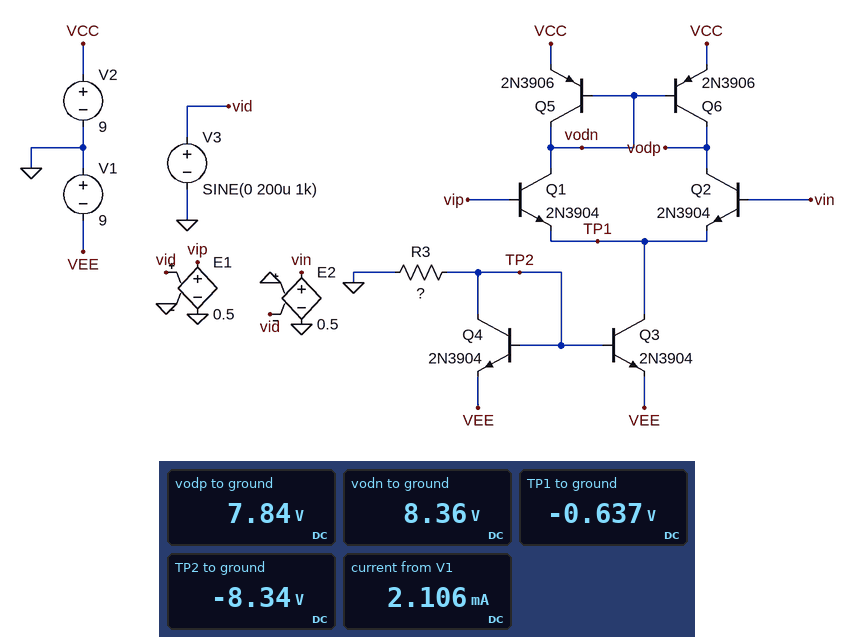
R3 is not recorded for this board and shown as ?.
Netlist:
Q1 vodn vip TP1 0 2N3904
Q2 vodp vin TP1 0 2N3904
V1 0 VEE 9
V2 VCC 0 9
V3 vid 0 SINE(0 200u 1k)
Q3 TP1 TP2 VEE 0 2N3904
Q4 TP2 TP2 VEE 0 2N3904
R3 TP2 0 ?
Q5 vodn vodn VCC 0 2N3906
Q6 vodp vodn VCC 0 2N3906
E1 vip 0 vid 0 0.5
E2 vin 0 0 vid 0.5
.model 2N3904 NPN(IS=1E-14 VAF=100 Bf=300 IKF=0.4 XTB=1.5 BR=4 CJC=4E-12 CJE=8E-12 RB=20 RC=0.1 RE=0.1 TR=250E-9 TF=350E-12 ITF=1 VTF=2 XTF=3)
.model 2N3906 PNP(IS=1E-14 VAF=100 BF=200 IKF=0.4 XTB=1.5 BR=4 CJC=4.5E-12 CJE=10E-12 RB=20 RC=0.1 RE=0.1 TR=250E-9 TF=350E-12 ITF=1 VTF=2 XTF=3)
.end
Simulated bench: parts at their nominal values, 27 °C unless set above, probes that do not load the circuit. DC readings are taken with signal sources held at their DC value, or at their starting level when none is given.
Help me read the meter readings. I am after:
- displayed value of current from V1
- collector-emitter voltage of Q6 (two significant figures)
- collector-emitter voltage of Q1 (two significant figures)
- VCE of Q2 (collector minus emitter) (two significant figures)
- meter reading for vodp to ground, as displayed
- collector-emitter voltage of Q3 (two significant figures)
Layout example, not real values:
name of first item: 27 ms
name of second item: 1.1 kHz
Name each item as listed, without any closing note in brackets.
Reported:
displayed value of current from V1: 2.106 mA
collector-emitter voltage of Q6: -1.2 V
collector-emitter voltage of Q1: 9.0 V
VCE of Q2 (collector minus emitter): 8.5 V
meter reading for vodp to ground, as displayed: 7.84 V
collector-emitter voltage of Q3: 8.4 V
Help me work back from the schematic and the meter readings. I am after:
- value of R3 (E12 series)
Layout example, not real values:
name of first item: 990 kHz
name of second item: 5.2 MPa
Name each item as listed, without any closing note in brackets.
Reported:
value of R3: 8.2 kΩ
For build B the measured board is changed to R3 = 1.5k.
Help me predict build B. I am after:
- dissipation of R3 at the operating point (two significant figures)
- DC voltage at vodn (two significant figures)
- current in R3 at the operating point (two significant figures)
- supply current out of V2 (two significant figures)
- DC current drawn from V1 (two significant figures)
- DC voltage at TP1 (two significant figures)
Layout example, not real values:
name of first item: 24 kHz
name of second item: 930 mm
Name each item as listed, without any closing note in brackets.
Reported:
dissipation of R3 at the operating point: 46 mW
DC voltage at vodn: 8.3 V
current in R3 at the operating point: 5.5 mA
supply current out of V2: 5.9 mA
DC current drawn from V1: 11 mA
DC voltage at TP1: -680 mV
